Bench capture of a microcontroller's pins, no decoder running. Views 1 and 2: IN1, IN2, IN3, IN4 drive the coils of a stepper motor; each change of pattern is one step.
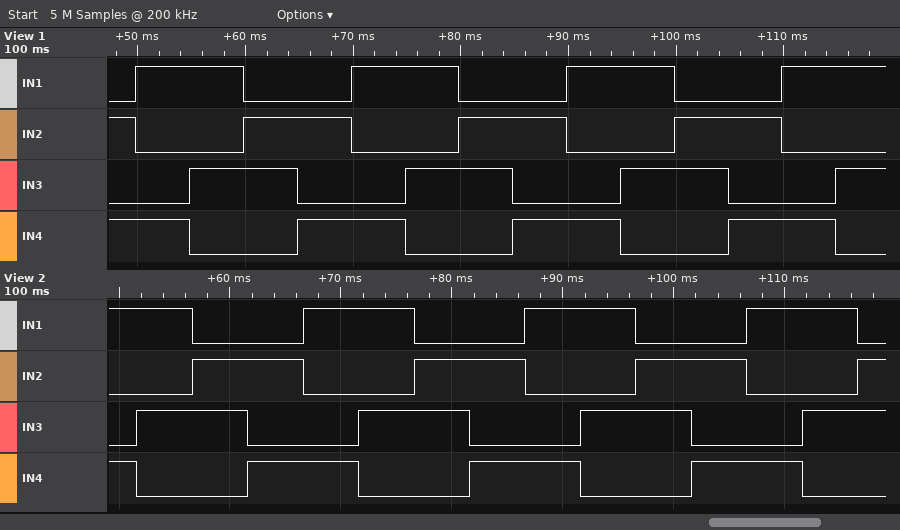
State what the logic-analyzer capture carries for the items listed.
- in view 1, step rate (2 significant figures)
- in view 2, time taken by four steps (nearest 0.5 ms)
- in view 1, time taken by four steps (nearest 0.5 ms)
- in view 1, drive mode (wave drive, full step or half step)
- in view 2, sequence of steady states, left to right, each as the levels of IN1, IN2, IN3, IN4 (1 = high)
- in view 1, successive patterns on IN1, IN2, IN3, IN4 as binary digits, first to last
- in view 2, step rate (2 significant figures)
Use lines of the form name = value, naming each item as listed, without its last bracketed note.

in view 1, step rate = 200 steps/s
in view 2, time taken by four steps = 20.0 ms
in view 1, time taken by four steps = 20.0 ms
in view 1, drive mode = full step
in view 2, sequence of steady states, left to right, each as the levels of IN1, IN2, IN3, IN4 = 1001 1010 0110 0101 1001 1010 0110 0101 1001 1010 0110 0101 1001 1010 0110
in view 1, successive patterns on IN1, IN2, IN3, IN4 as binary digits, first to last = 0101 1001 1010 0110 0101 1001 1010 0110 0101 1001 1010 0110 0101 1001 1010
in view 2, step rate = 200 steps/s
